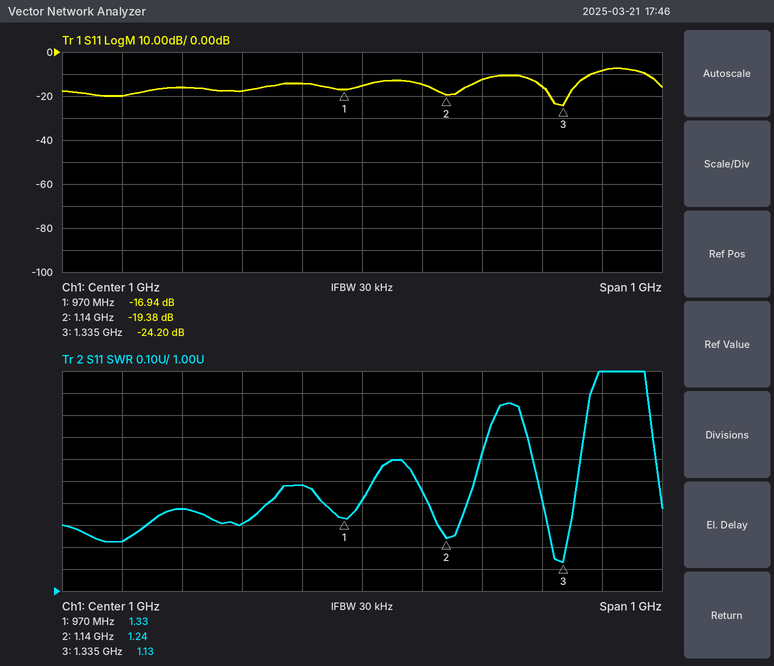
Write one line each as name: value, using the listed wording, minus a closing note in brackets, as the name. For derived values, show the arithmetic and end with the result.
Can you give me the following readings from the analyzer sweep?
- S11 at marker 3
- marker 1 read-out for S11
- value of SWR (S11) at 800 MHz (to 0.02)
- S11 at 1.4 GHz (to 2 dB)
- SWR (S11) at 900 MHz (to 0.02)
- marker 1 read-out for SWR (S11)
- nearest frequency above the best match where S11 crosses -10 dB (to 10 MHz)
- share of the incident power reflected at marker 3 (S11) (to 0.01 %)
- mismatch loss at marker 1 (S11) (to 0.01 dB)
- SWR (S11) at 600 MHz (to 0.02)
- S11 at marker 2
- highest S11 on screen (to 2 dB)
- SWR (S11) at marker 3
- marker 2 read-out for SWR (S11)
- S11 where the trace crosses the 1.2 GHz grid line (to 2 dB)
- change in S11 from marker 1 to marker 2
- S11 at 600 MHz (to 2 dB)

S11 at marker 3: -24.20 dB
marker 1 read-out for S11: -16.94 dB
value of SWR (S11) at 800 MHz: 1.30
S11 at 1.4 GHz: -8 dB
SWR (S11) at 900 MHz: 1.48
marker 1 read-out for SWR: 1.33
nearest frequency above the best match where S11 crosses -10 dB: 1.38 GHz
share of the incident power reflected at marker 3 (S11): 10^(-24.2/10) ≈ 0.38 %
mismatch loss at marker 1 (S11): −10 log10(1 − 10^(-16.94/10)) ≈ 0.09 dB
SWR (S11) at 600 MHz: 1.22
S11 at marker 2: -19.38 dB
highest S11 on screen: -8 dB
SWR (S11) at marker 3: 1.13
marker 2 read-out for SWR: 1.24
S11 where the trace crosses the 1.2 GHz grid line: -12 dB
change in S11 from marker 1 to marker 2: -19.38 − (-16.94) = -2.44 dB
S11 at 600 MHz: -20 dB
